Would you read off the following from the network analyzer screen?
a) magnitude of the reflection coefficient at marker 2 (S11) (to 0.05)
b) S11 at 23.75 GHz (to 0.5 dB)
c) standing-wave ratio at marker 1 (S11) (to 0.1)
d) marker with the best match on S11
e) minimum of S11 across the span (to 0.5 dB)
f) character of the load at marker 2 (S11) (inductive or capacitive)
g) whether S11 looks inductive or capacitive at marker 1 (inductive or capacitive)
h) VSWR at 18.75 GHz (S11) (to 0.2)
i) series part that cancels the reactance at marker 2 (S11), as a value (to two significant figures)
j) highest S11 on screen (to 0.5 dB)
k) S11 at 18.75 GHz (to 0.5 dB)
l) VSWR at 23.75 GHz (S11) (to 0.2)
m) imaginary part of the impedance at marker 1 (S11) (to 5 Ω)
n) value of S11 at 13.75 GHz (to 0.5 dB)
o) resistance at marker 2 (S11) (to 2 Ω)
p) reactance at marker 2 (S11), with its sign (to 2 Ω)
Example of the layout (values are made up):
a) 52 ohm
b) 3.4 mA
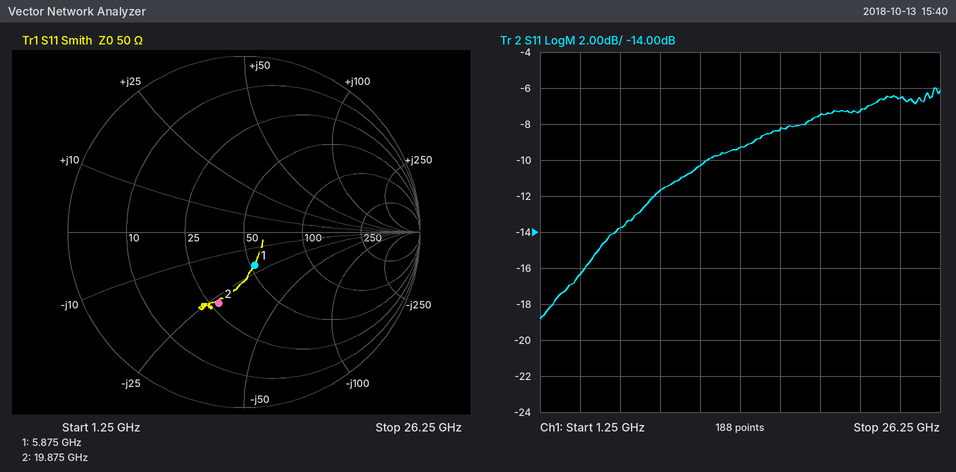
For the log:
a) 0.45
b) -6.5 dB
c) 1.5
d) marker 1
e) -19.0 dB
f) capacitive
g) capacitive
h) 2.4
i) 220 pH
j) -6.0 dB
k) -7.5 dB
l) 2.8
m) -20 Ω
n) -9.5 dB
o) 28 Ω
p) -28 Ω
